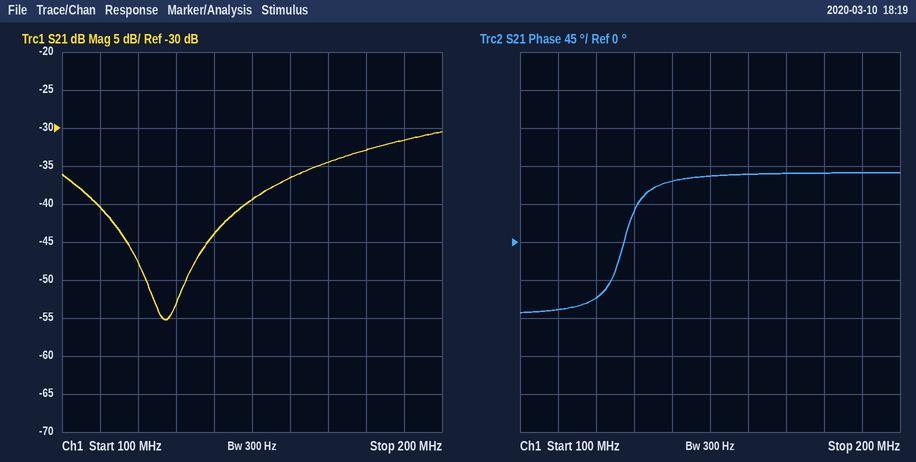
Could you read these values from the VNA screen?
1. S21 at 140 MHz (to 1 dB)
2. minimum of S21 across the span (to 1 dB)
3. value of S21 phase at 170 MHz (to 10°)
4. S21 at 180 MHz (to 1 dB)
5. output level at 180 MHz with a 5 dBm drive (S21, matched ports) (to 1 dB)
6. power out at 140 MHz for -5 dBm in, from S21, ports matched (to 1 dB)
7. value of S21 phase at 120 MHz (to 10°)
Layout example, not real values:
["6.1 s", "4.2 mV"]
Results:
["-44 dB", "-55 dB", "80°", "-33 dB", "-28 dBm", "-49 dBm", "-70°"]
